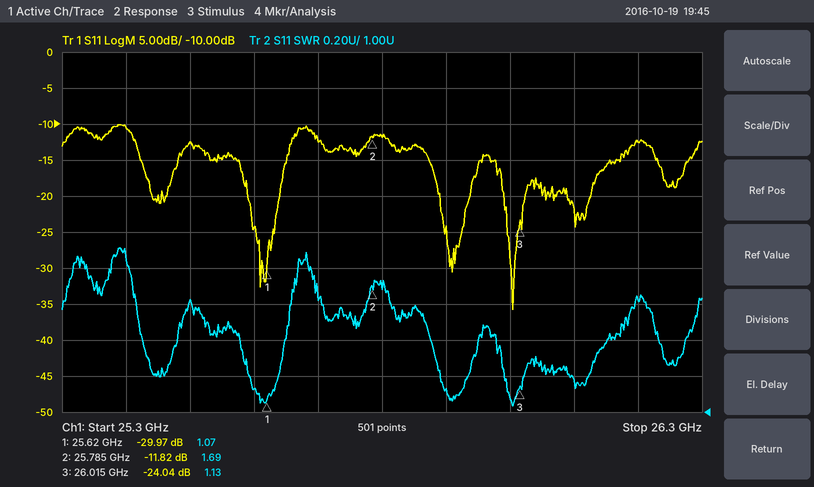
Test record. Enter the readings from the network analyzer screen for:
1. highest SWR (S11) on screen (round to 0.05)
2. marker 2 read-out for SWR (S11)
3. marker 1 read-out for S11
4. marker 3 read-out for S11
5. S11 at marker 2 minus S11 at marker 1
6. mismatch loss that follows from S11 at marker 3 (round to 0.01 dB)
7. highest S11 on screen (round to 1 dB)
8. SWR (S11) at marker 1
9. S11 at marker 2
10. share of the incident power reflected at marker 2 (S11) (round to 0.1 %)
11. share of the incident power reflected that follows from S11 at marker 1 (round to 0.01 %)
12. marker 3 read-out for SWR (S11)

1.90
1.69
-29.97 dB
-24.04 dB
18.15 dB
0.02 dB
-10 dB
1.07
-11.82 dB
6.6 %
0.10 %
1.13
